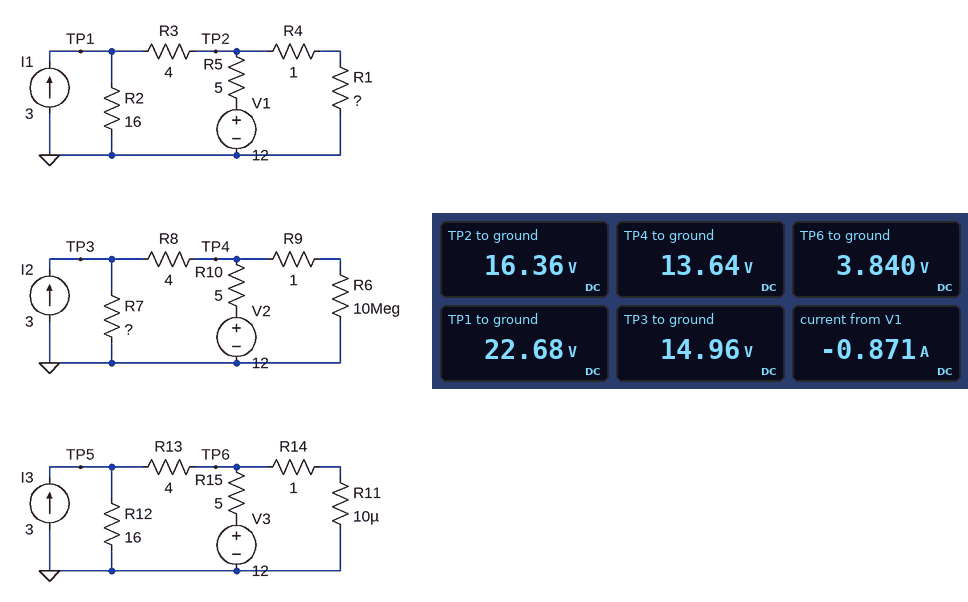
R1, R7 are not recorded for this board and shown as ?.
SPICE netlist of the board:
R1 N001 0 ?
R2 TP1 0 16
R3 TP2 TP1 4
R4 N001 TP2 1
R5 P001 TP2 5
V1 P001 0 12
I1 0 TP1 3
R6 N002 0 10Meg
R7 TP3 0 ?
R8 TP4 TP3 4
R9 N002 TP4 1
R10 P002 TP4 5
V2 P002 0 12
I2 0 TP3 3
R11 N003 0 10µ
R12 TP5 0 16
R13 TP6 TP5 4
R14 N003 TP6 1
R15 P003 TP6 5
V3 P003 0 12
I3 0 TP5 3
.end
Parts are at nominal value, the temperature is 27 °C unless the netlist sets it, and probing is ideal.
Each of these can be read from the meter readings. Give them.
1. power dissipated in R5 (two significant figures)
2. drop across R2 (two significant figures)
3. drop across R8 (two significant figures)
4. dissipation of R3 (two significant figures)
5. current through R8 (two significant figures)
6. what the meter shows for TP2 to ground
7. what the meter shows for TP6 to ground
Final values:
3.8 W
23 V
1.3 V
10 W
330 mA
16.36 V
3.840 V
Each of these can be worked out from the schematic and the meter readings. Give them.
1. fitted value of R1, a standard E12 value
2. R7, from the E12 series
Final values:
22 Ω
5.6 Ω
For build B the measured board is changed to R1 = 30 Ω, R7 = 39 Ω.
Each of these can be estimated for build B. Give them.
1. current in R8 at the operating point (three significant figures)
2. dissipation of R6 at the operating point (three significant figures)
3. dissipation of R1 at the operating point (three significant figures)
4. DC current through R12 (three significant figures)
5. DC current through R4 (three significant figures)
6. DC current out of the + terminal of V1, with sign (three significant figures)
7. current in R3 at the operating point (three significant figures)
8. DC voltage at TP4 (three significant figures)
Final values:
2.19 A
52.6 µW
9.03 W
792 mA
549 mA
-1.00 A
1.55 A
22.9 V
